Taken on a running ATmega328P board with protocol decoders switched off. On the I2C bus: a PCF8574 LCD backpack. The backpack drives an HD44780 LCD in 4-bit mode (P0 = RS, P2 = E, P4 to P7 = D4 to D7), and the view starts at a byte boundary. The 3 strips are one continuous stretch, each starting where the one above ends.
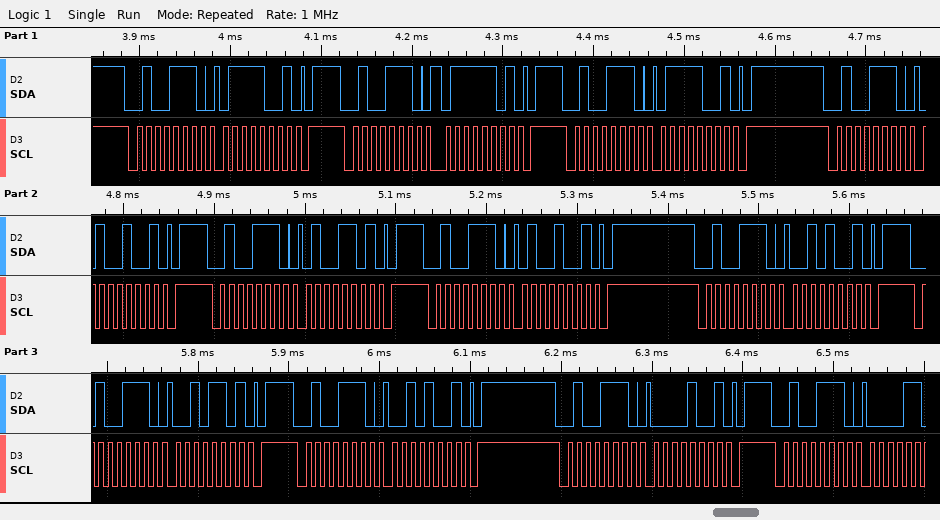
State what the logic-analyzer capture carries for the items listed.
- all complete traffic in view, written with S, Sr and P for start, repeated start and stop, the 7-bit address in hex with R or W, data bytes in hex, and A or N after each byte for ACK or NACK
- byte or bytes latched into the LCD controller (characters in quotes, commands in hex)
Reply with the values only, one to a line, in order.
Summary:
S 27W A 79 A P S 27W A 7D A P S 27W A 79 A P S 27W A 49 A P S 27W A 4D A P S 27W A 49 A P S 27W A 29 A P S 27W A 2D A P S 27W A 29 A P S 27W A 09 A P S 27W A
't'
